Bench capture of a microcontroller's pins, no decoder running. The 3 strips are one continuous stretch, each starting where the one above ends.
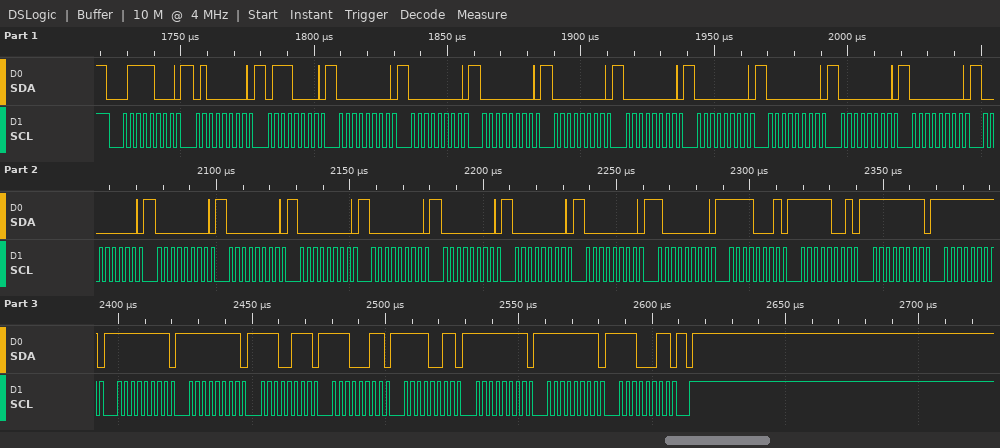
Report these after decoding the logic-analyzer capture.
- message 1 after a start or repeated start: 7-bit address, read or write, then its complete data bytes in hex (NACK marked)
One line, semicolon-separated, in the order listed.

0x3C write: 40 70 00 00 00 00 00 00 00 00 00 00 00 00 00 00 00 00 00 80 F1 F9 FF FF FF FF E7 E3 F3 FF FF E3
